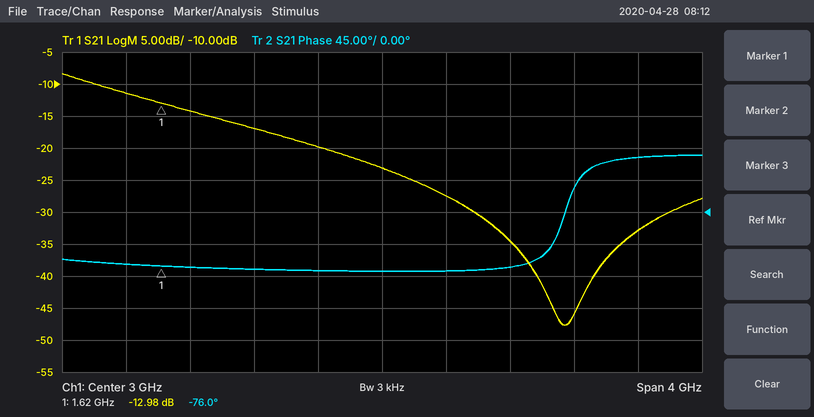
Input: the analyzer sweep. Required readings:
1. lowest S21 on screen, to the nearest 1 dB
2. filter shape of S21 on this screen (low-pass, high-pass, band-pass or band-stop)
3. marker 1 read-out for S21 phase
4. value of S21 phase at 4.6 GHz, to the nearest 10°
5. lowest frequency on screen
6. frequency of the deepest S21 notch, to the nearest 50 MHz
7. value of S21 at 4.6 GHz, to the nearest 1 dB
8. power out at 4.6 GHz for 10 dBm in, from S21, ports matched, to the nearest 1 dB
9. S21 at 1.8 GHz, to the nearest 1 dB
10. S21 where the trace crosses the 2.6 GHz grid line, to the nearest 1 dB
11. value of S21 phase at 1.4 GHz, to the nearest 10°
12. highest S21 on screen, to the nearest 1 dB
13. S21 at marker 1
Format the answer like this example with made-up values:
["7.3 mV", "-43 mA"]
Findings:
["-48 dB", "low-pass", "-76.0°", "80°", "1 GHz", "4.15 GHz", "-33 dB", "-23 dBm", "-14 dB", "-20 dB", "-70°", "-8 dB", "-12.98 dB"]
